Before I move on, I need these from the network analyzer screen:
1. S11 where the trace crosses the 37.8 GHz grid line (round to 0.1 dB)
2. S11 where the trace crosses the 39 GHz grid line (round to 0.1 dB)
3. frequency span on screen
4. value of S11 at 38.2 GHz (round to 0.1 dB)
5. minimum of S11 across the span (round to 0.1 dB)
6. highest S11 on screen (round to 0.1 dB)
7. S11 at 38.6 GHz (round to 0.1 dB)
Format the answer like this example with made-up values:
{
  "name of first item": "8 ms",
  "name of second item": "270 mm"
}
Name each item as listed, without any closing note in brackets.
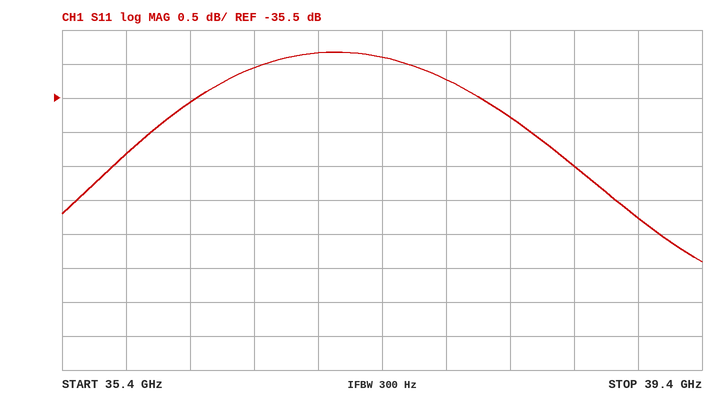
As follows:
{
  "S11 where the trace crosses the 37.8 GHz grid line": "-35.2 dB",
  "S11 where the trace crosses the 39 GHz grid line": "-37.3 dB",
  "frequency span on screen": "4 GHz",
  "value of S11 at 38.2 GHz": "-35.8 dB",
  "minimum of S11 across the span": "-37.9 dB",
  "highest S11 on screen": "-34.8 dB",
  "S11 at 38.6 GHz": "-36.5 dB"
}
